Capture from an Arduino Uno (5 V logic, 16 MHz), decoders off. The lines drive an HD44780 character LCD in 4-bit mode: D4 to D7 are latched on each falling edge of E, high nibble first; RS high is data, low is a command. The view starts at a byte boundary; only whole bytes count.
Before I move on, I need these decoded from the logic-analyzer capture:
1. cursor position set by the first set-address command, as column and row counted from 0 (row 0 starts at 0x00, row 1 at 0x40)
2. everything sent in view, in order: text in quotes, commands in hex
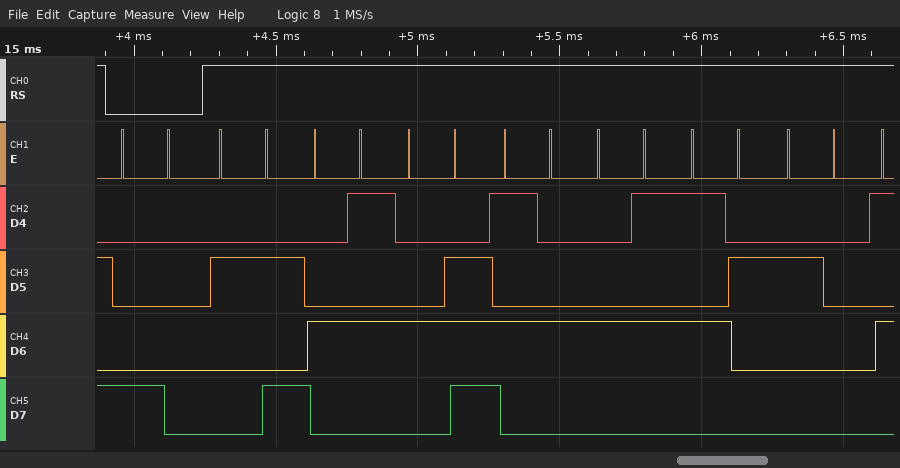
column 0, row 0
0x80 "*ENTER "
